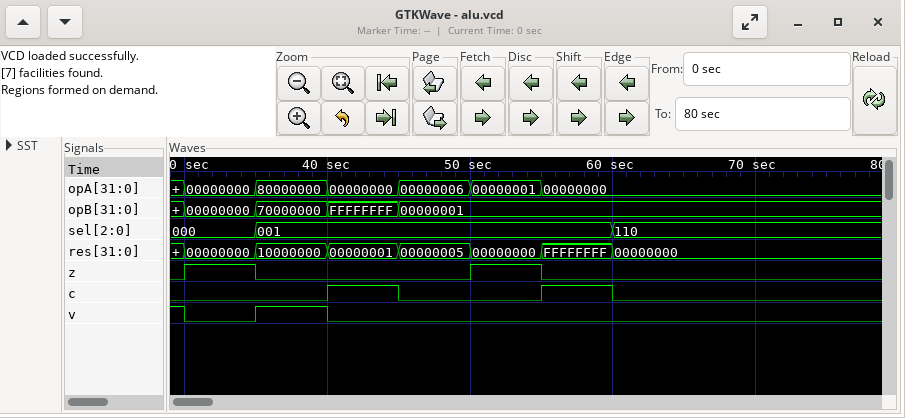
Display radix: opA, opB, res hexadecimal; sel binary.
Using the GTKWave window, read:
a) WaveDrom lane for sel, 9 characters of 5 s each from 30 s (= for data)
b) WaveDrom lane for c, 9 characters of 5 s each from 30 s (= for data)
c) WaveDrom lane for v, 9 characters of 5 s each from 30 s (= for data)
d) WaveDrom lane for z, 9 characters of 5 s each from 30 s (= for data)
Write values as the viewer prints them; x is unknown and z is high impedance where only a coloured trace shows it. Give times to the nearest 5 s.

{name: 'sel', wave: '==....=..', data: '000 001 110'}
{name: 'c', wave: '0.10.10..'}
{name: 'v', wave: '010......'}
{name: 'z', wave: '10..10...'}
